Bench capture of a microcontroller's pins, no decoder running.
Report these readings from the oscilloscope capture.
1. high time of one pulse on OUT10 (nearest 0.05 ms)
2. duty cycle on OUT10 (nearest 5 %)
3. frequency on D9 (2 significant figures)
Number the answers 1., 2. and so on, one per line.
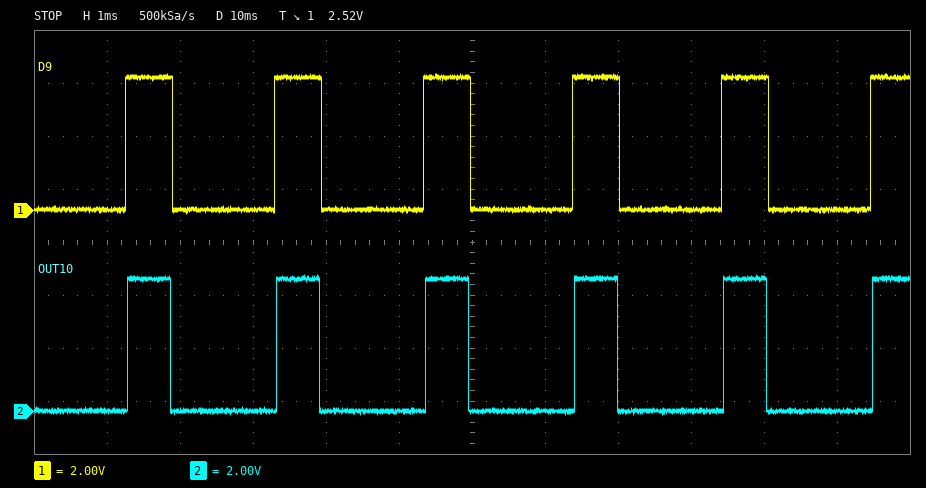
1. 0.60 ms
2. 30 %
3. 490 Hz
